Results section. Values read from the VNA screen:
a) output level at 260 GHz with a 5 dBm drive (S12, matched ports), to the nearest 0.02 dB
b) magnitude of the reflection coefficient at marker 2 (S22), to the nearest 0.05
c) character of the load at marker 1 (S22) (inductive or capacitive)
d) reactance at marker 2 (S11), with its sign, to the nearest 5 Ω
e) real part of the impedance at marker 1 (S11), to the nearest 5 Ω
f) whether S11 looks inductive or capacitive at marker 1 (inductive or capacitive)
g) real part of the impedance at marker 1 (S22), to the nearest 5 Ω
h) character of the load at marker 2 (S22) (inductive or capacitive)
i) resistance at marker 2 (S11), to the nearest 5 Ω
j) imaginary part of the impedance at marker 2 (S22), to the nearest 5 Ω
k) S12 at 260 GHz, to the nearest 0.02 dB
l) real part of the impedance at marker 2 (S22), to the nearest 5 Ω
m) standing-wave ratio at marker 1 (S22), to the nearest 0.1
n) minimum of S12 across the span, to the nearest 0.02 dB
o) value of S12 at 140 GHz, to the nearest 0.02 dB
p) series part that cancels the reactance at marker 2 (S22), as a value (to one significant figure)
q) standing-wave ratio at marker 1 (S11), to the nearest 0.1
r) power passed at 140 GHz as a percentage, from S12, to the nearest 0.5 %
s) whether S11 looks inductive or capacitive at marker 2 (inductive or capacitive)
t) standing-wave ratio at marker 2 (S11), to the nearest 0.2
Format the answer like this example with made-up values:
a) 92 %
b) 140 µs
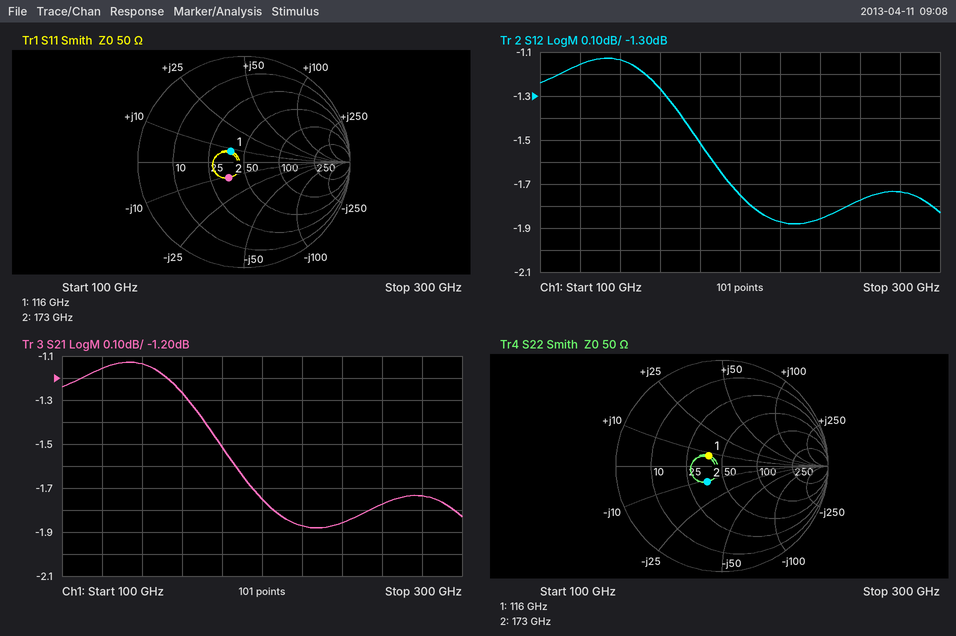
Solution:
a) 3.22 dBm
b) 0.20
c) inductive
d) -10 Ω
e) 40 Ω
f) inductive
g) 40 Ω
h) capacitive
i) 35 Ω
j) -10 Ω
k) -1.78 dB
l) 35 Ω
m) 1.4
n) -1.88 dB
o) -1.14 dB
p) 10 pH
q) 1.4
r) 77.0 %
s) capacitive
t) 1.6
